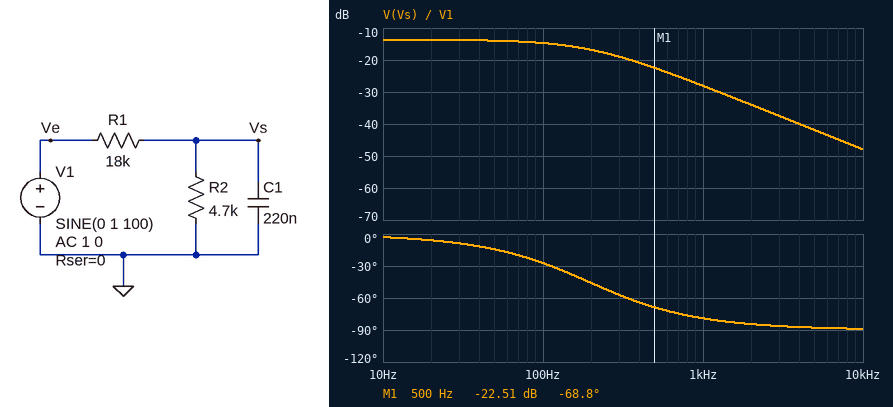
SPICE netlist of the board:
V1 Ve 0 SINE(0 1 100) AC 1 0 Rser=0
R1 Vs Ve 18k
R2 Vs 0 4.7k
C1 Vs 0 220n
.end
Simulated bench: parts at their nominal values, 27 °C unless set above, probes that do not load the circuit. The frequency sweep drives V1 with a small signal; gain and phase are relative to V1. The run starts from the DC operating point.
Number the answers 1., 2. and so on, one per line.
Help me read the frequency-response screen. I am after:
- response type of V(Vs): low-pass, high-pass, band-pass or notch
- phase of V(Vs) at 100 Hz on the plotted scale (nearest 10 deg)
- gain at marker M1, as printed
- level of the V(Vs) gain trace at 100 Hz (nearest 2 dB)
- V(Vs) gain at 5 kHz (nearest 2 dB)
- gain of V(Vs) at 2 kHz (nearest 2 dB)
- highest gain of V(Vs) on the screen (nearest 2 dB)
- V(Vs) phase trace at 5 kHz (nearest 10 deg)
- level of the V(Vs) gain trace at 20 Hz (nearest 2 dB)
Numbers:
1. low-pass
2. -30 deg
3. -22.51 dB
4. -14 dB
5. -42 dB
6. -34 dB
7. -14 dB
8. -90 deg
9. -14 dB
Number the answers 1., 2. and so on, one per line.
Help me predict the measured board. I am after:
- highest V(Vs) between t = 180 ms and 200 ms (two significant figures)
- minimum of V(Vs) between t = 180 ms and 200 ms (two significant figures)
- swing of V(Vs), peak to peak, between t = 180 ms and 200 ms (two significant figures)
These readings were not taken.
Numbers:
1. 180 mV
2. -180 mV
3. 370 mV
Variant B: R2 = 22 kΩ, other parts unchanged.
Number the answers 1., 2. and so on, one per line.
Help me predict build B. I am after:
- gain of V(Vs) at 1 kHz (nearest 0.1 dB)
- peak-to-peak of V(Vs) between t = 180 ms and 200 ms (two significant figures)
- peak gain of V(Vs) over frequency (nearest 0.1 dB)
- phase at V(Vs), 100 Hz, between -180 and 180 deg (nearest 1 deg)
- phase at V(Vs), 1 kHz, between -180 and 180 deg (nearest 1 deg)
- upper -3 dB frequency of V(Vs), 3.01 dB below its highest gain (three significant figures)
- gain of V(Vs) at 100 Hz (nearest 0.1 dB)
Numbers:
1. -27.9 dB
2. 650 mV
3. -5.2 dB
4. -54 deg
5. -86 deg
6. 73.1 Hz
7. -9.8 dB
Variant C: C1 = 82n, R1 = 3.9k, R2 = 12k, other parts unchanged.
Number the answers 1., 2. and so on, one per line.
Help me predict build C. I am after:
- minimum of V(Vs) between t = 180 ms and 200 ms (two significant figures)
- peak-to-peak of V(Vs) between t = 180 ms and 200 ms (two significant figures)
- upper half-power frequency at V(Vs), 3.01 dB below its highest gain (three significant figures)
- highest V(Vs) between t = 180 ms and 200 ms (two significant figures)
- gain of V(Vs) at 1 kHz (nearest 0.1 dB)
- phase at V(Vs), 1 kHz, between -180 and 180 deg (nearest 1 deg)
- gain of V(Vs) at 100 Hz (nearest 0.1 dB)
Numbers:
1. -750 mV
2. 1.5 V
3. 659 Hz
4. 750 mV
5. -7.6 dB
6. -57 deg
7. -2.5 dB
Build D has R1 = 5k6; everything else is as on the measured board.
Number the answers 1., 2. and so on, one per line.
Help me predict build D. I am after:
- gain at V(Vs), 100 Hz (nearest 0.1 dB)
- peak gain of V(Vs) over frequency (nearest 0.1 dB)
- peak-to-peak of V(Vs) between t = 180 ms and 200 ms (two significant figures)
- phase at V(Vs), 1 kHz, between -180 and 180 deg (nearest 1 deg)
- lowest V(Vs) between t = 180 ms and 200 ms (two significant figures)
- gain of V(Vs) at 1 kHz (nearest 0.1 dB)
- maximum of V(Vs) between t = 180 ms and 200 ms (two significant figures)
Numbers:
1. -7.3 dB
2. -6.8 dB
3. 860 mV
4. -74 deg
5. -430 mV
6. -18.1 dB
7. 430 mV
